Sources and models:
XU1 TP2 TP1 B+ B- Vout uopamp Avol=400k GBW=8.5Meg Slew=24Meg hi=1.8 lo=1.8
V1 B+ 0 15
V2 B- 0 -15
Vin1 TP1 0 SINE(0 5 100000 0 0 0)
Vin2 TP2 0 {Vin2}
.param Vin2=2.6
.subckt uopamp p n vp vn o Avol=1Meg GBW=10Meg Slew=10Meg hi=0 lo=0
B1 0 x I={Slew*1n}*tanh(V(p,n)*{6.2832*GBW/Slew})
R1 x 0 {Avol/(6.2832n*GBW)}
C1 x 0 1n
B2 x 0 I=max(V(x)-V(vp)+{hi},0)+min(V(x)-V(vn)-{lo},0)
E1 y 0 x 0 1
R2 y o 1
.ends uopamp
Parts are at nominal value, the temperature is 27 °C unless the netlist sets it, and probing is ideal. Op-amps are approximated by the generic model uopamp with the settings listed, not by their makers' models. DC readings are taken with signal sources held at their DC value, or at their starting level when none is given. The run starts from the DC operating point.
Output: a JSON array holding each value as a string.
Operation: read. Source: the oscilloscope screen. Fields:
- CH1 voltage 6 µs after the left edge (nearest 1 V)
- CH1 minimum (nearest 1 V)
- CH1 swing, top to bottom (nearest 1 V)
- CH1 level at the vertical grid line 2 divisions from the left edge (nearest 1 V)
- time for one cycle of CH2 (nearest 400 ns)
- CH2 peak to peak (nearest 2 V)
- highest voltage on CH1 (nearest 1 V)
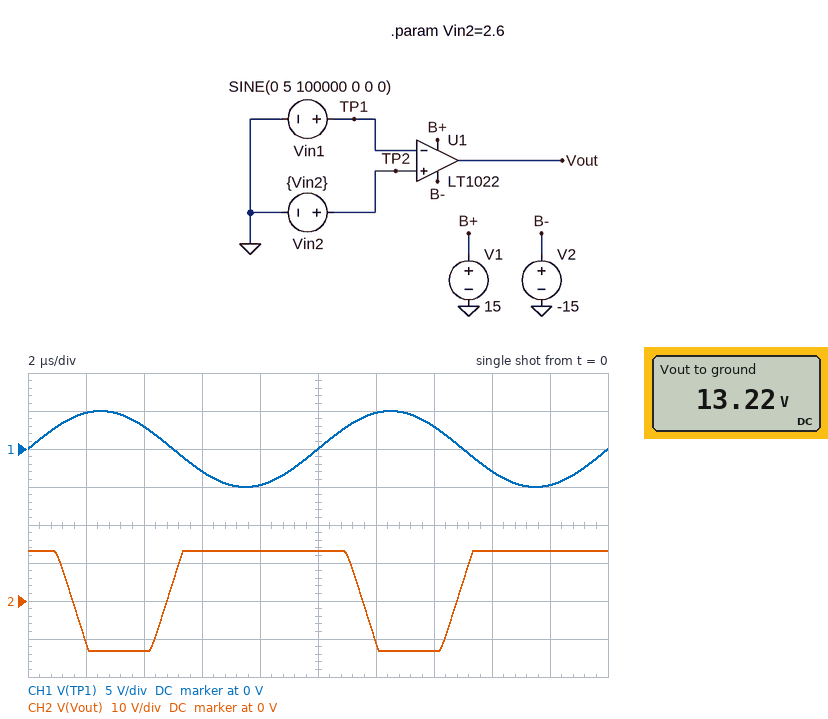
["-3 V", "-5 V", "10 V", "3 V", "10.0 µs", "26 V", "5 V"]
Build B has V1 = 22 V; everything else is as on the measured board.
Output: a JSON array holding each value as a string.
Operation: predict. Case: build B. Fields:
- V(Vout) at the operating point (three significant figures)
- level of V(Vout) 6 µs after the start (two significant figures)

["20.2 V", "20 V"]
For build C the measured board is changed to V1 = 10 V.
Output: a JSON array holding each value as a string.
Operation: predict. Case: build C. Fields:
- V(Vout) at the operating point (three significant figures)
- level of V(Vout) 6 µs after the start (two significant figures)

["8.22 V", "8.2 V"]
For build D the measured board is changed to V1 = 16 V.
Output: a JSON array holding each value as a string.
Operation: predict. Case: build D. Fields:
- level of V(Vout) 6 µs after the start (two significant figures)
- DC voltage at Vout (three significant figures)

["14 V", "14.2 V"]
